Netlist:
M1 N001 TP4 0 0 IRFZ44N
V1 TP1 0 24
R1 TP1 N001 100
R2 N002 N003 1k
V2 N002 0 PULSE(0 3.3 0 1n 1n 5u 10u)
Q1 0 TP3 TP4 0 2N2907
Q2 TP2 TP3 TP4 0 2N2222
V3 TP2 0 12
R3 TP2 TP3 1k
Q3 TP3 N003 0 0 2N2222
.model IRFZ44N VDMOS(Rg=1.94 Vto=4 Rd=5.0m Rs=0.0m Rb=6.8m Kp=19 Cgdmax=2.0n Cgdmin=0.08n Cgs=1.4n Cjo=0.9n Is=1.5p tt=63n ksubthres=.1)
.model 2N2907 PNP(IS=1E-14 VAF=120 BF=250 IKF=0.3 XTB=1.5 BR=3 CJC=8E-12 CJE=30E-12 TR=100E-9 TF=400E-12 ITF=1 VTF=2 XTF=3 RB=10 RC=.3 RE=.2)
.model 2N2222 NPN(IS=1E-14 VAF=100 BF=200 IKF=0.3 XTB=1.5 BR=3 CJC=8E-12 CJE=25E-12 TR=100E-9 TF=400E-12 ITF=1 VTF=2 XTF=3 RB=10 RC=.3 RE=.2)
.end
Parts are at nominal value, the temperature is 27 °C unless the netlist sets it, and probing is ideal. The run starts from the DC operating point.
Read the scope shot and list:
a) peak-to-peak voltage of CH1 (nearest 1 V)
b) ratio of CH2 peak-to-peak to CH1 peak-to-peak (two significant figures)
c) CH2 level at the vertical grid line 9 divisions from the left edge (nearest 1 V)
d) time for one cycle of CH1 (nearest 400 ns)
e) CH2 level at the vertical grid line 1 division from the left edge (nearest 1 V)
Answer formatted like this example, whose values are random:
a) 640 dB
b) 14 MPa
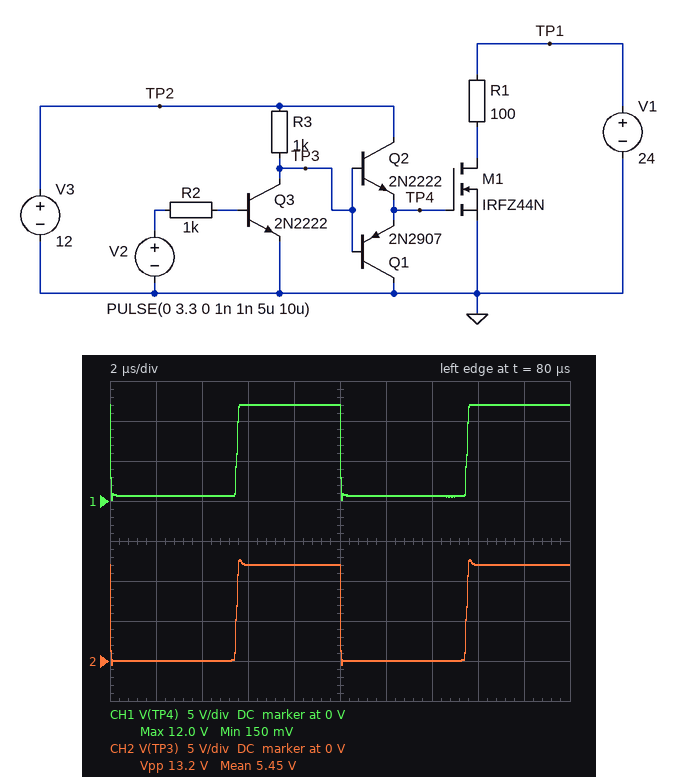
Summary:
a) 12 V
b) 1.1
c) 12 V
d) 10.0 µs
e) 0 V
